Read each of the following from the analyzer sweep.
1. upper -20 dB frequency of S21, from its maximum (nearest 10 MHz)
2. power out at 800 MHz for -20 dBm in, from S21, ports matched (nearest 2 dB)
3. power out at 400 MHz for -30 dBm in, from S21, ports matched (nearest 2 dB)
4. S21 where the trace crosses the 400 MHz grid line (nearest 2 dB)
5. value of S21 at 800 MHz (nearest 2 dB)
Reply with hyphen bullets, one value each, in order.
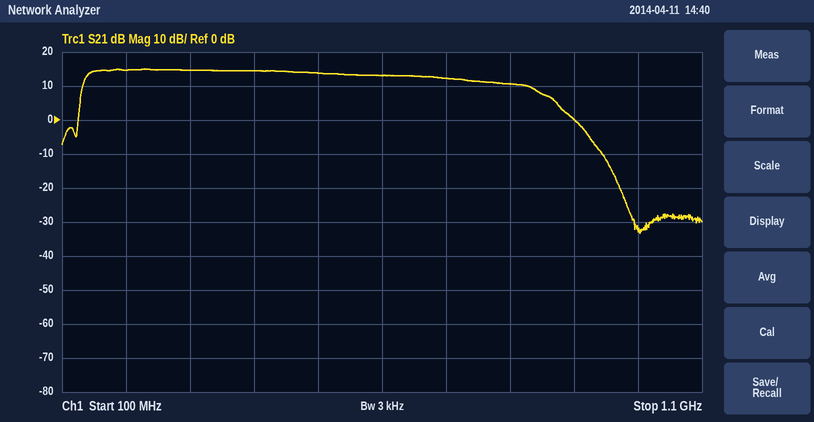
- 920 MHz
- -10 dBm
- -16 dBm
- 14 dB
- 10 dB
